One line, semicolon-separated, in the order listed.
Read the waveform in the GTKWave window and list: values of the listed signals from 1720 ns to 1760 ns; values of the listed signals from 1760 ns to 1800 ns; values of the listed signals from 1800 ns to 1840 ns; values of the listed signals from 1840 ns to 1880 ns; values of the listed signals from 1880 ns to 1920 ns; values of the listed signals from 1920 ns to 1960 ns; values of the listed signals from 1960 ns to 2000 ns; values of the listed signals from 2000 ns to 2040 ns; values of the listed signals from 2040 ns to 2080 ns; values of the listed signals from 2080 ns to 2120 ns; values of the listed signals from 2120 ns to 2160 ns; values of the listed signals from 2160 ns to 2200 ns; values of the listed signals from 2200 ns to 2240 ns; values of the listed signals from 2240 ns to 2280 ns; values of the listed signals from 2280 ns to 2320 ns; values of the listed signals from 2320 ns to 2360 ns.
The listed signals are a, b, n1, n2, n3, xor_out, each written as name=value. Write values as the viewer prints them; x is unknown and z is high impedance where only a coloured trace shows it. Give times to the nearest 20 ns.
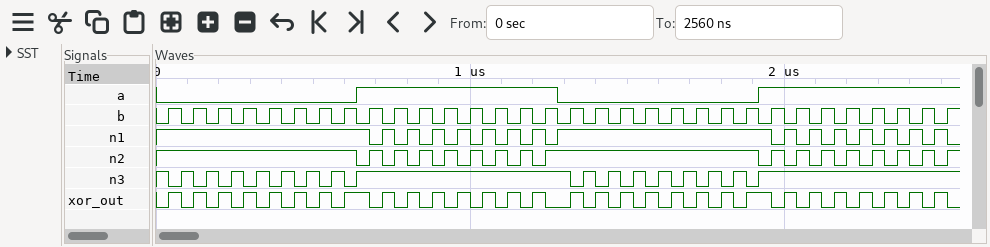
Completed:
a=0, b=1, n1=1, n2=1, n3=0, xor_out=1; a=0, b=0, n1=1, n2=1, n3=1, xor_out=0; a=0, b=1, n1=1, n2=1, n3=0, xor_out=1; a=0, b=0, n1=1, n2=1, n3=1, xor_out=0; a=0, b=1, n1=1, n2=1, n3=0, xor_out=1; a=1, b=0, n1=1, n2=0, n3=1, xor_out=1; a=1, b=1, n1=0, n2=1, n3=1, xor_out=0; a=1, b=0, n1=1, n2=0, n3=1, xor_out=1; a=1, b=1, n1=0, n2=1, n3=1, xor_out=0; a=1, b=0, n1=1, n2=0, n3=1, xor_out=1; a=1, b=1, n1=0, n2=1, n3=1, xor_out=0; a=1, b=0, n1=1, n2=0, n3=1, xor_out=1; a=1, b=1, n1=0, n2=1, n3=1, xor_out=0; a=1, b=0, n1=1, n2=0, n3=1, xor_out=1; a=1, b=1, n1=0, n2=1, n3=1, xor_out=0; a=1, b=0, n1=1, n2=0, n3=1, xor_out=1
